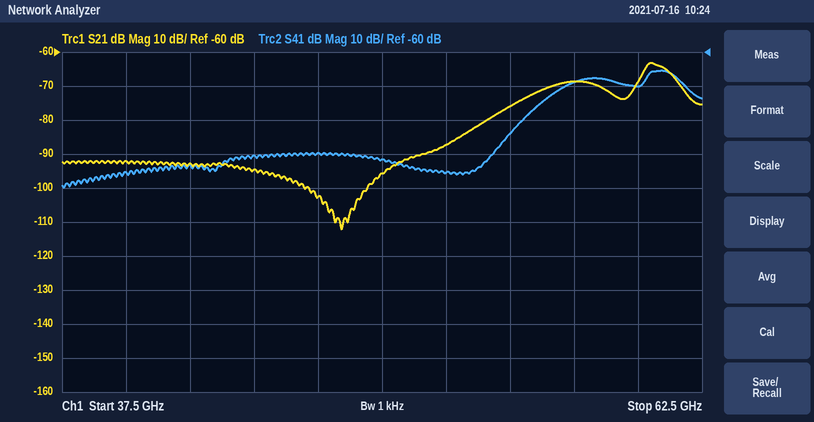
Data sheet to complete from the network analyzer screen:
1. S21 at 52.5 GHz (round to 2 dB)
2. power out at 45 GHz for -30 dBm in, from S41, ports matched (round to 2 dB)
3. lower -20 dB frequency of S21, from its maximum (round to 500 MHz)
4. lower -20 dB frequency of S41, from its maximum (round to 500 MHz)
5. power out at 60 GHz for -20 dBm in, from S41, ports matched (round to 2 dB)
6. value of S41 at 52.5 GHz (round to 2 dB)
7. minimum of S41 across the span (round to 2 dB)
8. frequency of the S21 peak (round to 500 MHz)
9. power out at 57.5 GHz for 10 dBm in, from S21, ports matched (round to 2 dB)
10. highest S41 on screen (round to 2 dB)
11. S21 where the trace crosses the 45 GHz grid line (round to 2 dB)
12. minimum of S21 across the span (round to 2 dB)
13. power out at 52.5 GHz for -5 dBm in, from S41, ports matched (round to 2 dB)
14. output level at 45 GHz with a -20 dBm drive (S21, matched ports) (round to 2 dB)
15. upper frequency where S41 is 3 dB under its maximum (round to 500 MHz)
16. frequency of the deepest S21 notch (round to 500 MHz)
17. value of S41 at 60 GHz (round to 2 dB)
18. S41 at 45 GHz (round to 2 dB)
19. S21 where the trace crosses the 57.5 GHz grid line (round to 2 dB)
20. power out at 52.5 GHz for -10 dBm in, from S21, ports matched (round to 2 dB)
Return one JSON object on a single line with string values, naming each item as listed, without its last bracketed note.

{"S21 at 52.5 GHz": "-88 dB", "power out at 45 GHz for -30 dBm in, from S41, ports matched": "-120 dBm", "lower -20 dB frequency of S21, from its maximum": "53.5 GHz", "lower -20 dB frequency of S41, from its maximum": "55.0 GHz", "power out at 60 GHz for -20 dBm in, from S41, ports matched": "-90 dBm", "value of S41 at 52.5 GHz": "-96 dB", "minimum of S41 across the span": "-100 dB", "frequency of the S21 peak": "60.5 GHz", "power out at 57.5 GHz for 10 dBm in, from S21, ports matched": "-58 dBm", "highest S41 on screen": "-66 dB", "S21 where the trace crosses the 45 GHz grid line": "-94 dB", "minimum of S21 across the span": "-112 dB", "power out at 52.5 GHz for -5 dBm in, from S41, ports matched": "-100 dBm", "output level at 45 GHz with a -20 dBm drive (S21, matched ports)": "-114 dBm", "upper frequency where S41 is 3 dB under its maximum": "61.5 GHz", "frequency of the deepest S21 notch": "48.5 GHz", "value of S41 at 60 GHz": "-70 dB", "S41 at 45 GHz": "-90 dB", "S21 where the trace crosses the 57.5 GHz grid line": "-68 dB", "power out at 52.5 GHz for -10 dBm in, from S21, ports matched": "-98 dBm"}
